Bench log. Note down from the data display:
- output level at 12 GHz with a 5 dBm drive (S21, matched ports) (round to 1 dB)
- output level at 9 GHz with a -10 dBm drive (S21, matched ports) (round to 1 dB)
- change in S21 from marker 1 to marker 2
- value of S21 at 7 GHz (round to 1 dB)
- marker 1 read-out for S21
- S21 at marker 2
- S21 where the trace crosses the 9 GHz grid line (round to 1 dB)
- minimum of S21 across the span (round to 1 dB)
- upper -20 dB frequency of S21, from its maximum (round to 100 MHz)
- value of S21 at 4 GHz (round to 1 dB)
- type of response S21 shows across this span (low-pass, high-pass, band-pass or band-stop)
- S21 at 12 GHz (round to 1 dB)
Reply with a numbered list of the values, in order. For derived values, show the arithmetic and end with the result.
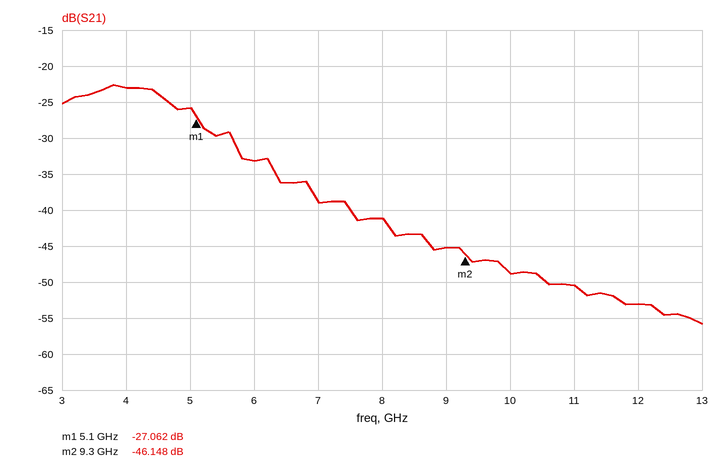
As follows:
1. 5 dBm + (-53 dB) = -48 dBm
2. -10 dBm + (-45 dB) = -55 dBm
3. -46.148 − (-27.062) = -19.086 dB
4. -39 dB
5. -27.062 dB
6. -46.148 dB
7. -45 dB
8. -56 dB
9. 8.1 GHz
10. -23 dB
11. low-pass
12. -53 dB
